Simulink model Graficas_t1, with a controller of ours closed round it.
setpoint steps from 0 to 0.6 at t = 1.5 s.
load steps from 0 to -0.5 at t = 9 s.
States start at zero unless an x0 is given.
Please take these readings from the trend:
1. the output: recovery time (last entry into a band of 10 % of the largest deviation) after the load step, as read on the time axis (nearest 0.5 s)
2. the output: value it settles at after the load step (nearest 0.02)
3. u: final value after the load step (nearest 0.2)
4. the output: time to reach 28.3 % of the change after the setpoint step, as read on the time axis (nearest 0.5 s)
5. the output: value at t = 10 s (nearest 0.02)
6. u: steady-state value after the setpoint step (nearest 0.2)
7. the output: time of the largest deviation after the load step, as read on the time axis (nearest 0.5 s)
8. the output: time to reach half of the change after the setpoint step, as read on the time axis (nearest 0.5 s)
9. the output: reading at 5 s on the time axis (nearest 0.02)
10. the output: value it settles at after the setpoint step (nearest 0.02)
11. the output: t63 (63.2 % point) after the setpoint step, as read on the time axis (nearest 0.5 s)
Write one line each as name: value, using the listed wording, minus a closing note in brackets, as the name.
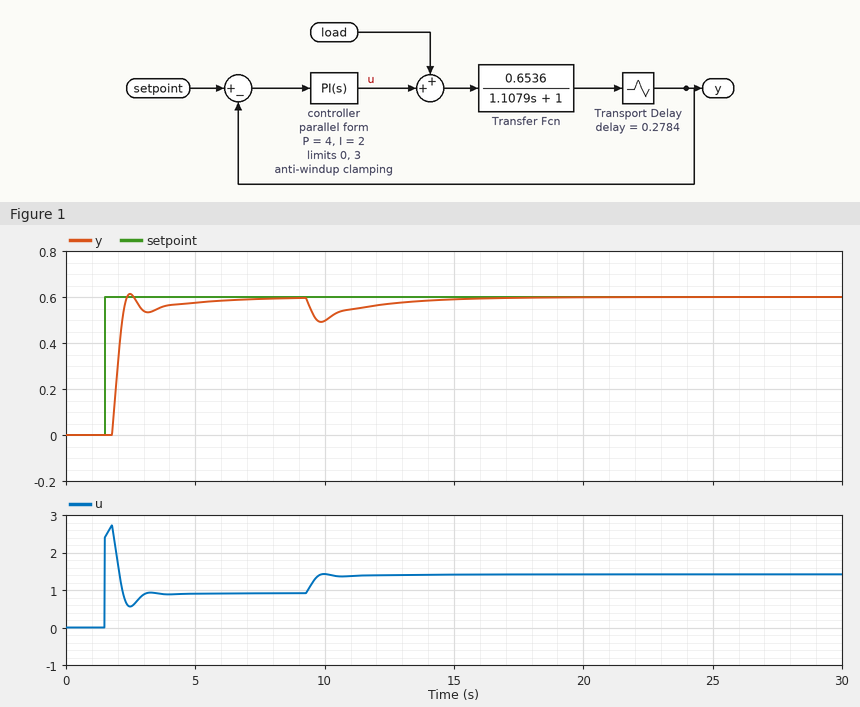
the output: recovery time (last entry into a band of 10 % of the largest deviation) after the load step, as read on the time axis: 15.0 s
the output: value it settles at after the load step: 0.60
u: final value after the load step: 1.4
the output: time to reach 28.3 % of the change after the setpoint step, as read on the time axis: 2.0 s
the output: value at t = 10 s: 0.50
u: steady-state value after the setpoint step: 1.0
the output: time of the largest deviation after the load step, as read on the time axis: 10.0 s
the output: time to reach half of the change after the setpoint step, as read on the time axis: 2.0 s
the output: reading at 5 s on the time axis: 0.58
the output: value it settles at after the setpoint step: 0.60
the output: t63 (63.2 % point) after the setpoint step, as read on the time axis: 2.0 s
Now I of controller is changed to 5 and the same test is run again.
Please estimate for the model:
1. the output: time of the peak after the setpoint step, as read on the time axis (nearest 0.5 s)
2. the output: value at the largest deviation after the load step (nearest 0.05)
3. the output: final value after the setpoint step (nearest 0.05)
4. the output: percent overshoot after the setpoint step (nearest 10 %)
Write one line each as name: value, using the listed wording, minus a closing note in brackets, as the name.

the output: time of the peak after the setpoint step, as read on the time axis: 2.5 s
the output: value at the largest deviation after the load step: 0.50
the output: final value after the setpoint step: 0.60
the output: percent overshoot after the setpoint step: 20 %
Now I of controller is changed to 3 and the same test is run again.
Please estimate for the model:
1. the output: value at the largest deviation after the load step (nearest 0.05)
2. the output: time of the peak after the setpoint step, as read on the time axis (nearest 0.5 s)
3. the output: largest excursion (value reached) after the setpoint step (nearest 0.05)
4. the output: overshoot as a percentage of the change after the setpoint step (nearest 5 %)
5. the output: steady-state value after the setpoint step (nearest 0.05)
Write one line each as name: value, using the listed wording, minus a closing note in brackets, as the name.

the output: value at the largest deviation after the load step: 0.50
the output: time of the peak after the setpoint step, as read on the time axis: 2.5 s
the output: largest excursion (value reached) after the setpoint step: 0.65
the output: overshoot as a percentage of the change after the setpoint step: 10 %
the output: steady-state value after the setpoint step: 0.60
